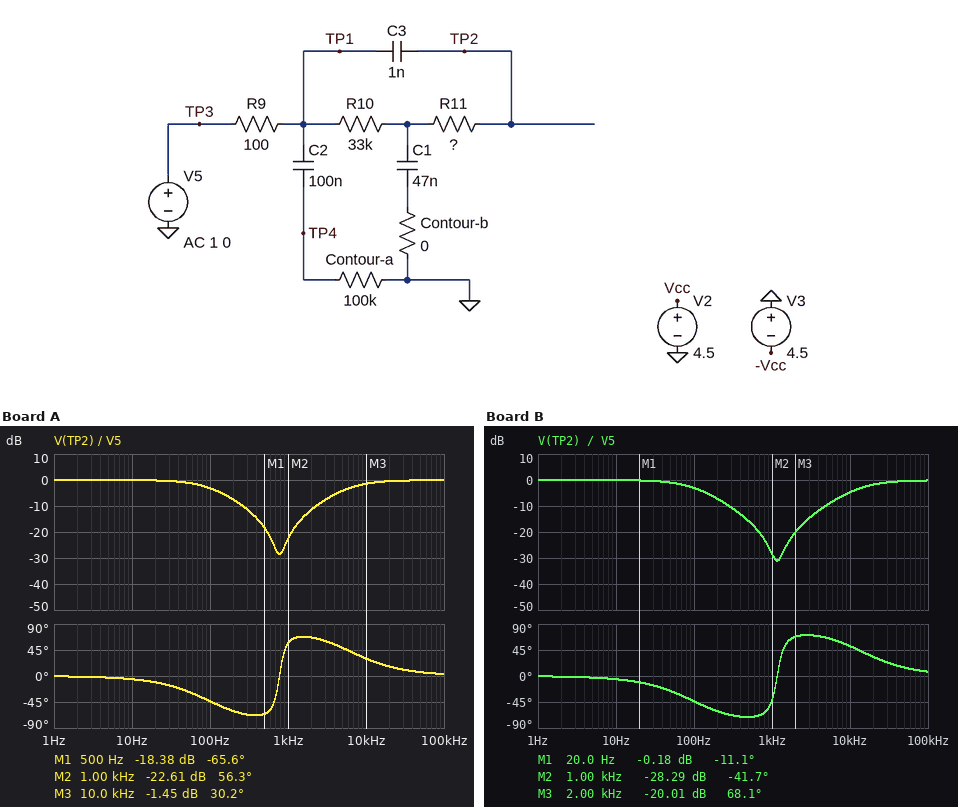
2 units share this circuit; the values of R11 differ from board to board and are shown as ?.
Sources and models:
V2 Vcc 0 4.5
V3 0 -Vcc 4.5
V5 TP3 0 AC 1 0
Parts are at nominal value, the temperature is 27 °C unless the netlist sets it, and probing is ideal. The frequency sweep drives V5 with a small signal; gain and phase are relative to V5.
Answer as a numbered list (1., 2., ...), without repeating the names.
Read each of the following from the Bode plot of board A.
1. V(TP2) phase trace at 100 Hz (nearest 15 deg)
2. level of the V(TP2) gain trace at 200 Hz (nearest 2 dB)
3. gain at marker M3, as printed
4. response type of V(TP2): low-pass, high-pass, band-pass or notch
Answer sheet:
1. -45 deg
2. -8 dB
3. -1.45 dB
4. notch
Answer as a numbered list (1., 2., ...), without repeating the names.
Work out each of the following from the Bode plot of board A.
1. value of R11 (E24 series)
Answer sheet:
1. 27 kΩ
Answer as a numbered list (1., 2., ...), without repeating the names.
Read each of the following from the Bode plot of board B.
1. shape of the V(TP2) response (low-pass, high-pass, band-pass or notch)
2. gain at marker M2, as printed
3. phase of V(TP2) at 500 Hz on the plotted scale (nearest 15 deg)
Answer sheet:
1. notch
2. -28.29 dB
3. -75 deg
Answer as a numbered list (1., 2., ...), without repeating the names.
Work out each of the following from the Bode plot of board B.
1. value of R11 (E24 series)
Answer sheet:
1. 12 kΩ
